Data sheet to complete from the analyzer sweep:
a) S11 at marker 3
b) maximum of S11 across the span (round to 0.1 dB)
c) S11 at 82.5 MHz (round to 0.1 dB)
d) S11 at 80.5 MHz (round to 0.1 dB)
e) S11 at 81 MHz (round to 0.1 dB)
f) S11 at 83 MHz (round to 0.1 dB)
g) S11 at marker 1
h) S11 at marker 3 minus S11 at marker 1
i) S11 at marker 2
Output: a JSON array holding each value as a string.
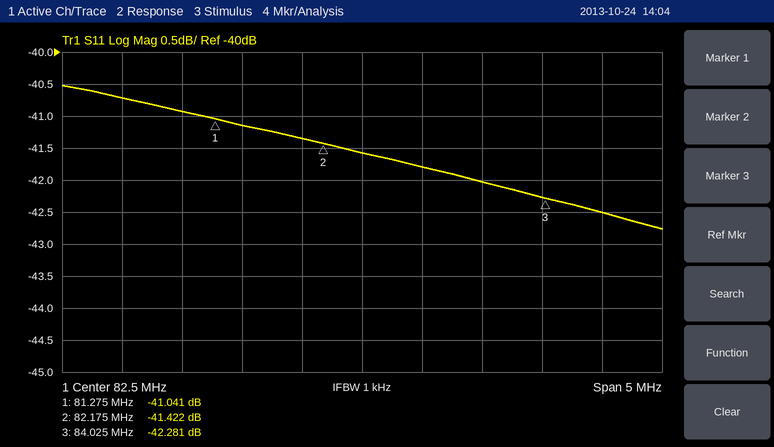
["-42.281 dB", "-40.5 dB", "-41.6 dB", "-40.7 dB", "-40.9 dB", "-41.8 dB", "-41.041 dB", "-1.240 dB", "-41.422 dB"]
